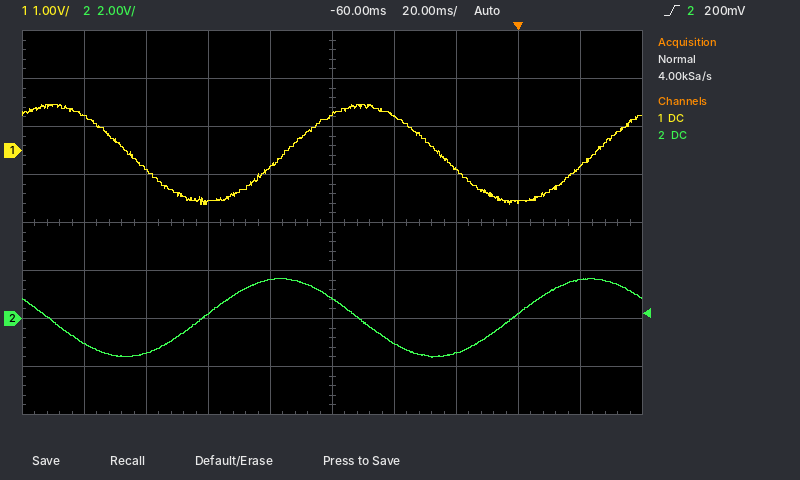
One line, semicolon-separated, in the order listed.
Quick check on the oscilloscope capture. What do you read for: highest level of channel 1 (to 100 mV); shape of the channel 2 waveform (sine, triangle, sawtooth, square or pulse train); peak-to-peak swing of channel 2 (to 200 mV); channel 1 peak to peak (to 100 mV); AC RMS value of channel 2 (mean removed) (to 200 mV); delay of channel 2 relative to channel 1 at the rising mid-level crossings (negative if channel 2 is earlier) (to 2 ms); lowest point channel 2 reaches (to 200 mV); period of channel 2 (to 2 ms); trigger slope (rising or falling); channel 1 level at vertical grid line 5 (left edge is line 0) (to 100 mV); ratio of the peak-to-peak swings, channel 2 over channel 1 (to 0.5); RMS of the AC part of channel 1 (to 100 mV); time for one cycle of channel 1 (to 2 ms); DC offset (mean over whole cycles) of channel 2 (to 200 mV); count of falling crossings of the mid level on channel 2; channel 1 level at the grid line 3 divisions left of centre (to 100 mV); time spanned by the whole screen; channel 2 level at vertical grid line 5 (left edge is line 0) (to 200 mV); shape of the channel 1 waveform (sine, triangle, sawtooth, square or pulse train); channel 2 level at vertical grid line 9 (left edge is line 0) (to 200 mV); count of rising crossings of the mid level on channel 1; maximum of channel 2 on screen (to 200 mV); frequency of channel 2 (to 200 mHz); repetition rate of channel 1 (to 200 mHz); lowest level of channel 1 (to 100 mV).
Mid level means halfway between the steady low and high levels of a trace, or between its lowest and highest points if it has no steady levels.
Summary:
1.0 V; sine; 3.2 V; 2.1 V; 1.2 V; -26 ms; -1.6 V; 100 ms; rising; 700 mV; 1.5; 700 mV; 100 ms; 0.0 V; 2; -400 mV; 200 ms; 800 mV; sine; 1.6 V; 2; 1.6 V; 10.0 Hz; 10.0 Hz; -1.1 V
